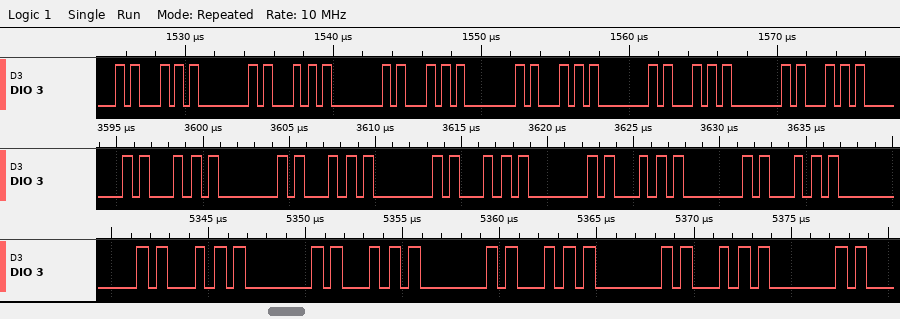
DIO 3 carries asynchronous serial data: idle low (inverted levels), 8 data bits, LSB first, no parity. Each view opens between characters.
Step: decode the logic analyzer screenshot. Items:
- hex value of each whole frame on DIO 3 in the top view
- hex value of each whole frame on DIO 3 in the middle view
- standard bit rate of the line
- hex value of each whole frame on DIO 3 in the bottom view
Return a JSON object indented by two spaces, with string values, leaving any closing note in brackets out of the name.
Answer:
{
  "hex value of each whole frame on DIO 3 in the top view": "5D, 7F, 57, 5D, 7F, 57, 5D, 7F, 57",
  "hex value of each whole frame on DIO 3 in the middle view": "5D, 7F, 57, 5D, 7F, 57, 5D",
  "standard bit rate of the line": "2000000 baud",
  "hex value of each whole frame on DIO 3 in the bottom view": "5D, 7F, 57, 5D, 7F, 57"
}
